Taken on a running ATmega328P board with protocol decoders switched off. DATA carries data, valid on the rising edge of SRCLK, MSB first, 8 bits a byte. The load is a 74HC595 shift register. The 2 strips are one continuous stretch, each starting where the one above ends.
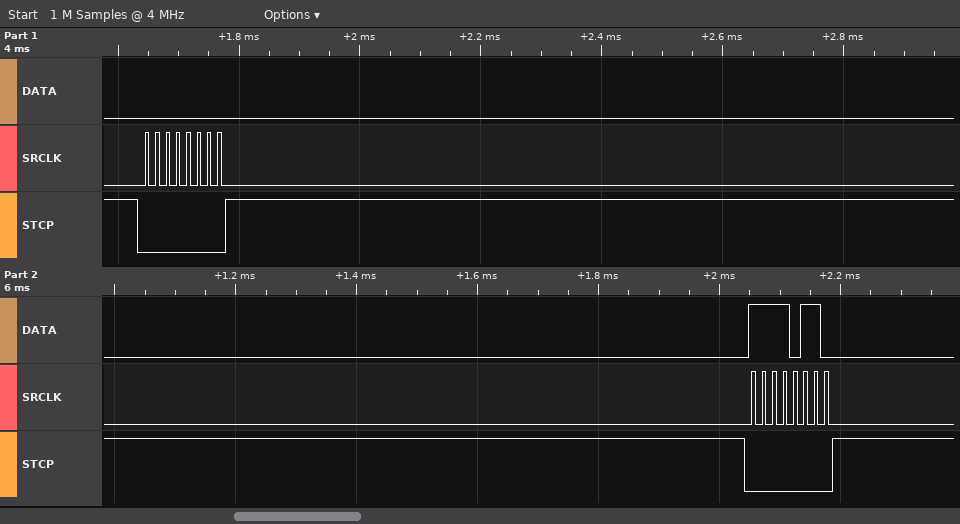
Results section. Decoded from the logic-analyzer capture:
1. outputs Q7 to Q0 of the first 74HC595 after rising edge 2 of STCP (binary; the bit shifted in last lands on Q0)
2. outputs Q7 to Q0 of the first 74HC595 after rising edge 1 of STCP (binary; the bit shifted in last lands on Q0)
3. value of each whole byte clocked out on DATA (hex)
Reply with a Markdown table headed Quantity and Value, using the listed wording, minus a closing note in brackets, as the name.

| Quantity | Value |
|---|---|
| outputs Q7 to Q0 of the first 74HC595 after rising edge 2 of STCP | 11110110 |
| outputs Q7 to Q0 of the first 74HC595 after rising edge 1 of STCP | 00000000 |
| value of each whole byte clocked out on DATA | 00 F6 |
